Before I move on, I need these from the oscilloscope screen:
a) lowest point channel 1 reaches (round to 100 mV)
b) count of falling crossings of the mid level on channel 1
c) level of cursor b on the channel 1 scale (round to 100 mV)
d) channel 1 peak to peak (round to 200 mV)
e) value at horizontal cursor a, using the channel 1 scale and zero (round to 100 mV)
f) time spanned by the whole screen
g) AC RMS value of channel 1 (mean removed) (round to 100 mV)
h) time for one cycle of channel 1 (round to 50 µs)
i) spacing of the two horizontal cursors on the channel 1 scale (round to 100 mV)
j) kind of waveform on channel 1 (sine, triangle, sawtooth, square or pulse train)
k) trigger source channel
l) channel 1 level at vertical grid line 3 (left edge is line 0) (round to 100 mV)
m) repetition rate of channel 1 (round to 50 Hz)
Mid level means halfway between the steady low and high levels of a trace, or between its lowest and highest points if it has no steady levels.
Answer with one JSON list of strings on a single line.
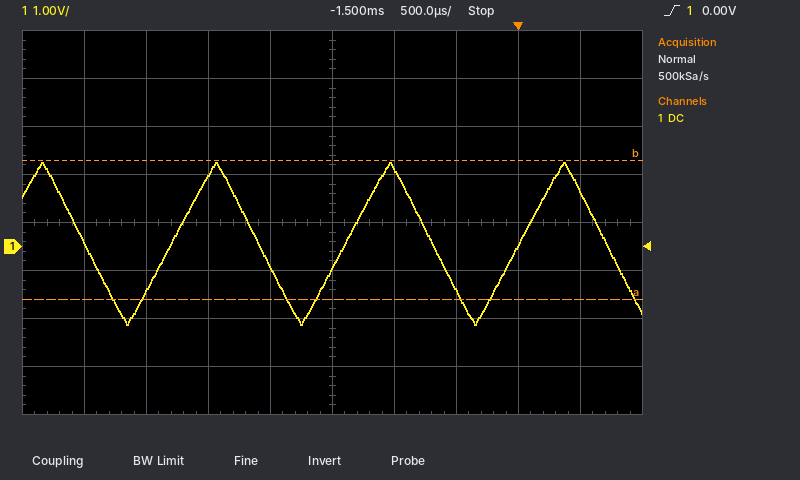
["-1.6 V", "4", "1.8 V", "3.4 V", "-1.1 V", "5 ms", "1.0 V", "1.40 ms", "2.9 V", "triangle", "channel 1", "1.5 V", "700 Hz"]
